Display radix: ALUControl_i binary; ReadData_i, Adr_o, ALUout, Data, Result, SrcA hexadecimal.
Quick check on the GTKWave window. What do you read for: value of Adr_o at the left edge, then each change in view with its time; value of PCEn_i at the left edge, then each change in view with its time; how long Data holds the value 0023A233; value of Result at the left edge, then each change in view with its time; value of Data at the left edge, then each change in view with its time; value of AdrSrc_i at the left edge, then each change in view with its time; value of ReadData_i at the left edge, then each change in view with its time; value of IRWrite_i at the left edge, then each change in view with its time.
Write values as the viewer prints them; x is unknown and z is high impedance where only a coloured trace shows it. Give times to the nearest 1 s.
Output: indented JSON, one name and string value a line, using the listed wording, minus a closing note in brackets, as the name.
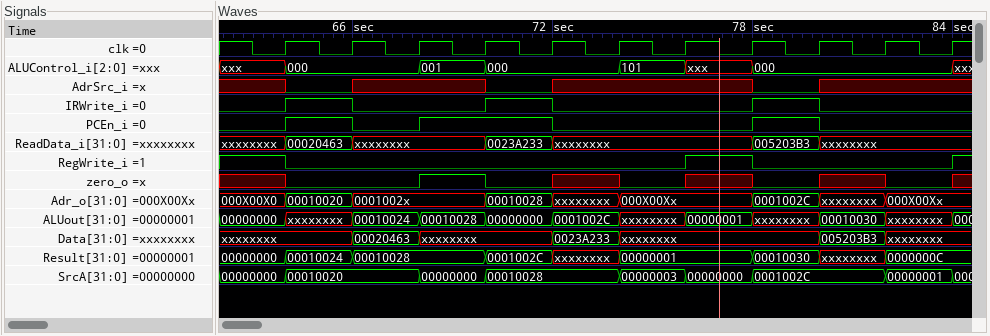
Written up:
{
  "value of Adr_o at the left edge, then each change in view with its time": "000X00X0, 00010020 at 64 s, 0001002x at 66 s, 00010028 at 70 s, xxxxxxxx at 72 s, 000X00Xx at 74 s, 0001002C at 78 s, xxxxxxxx at 80 s, 000X00Xx at 82 s",
  "value of PCEn_i at the left edge, then each change in view with its time": "0, 1 at 64 s, 0 at 66 s, 1 at 68 s, 0 at 72 s, 1 at 78 s, 0 at 80 s",
  "how long Data holds the value 0023A233": "2 s",
  "value of Result at the left edge, then each change in view with its time": "00000000, 00010024 at 64 s, 00010028 at 66 s, 0001002C at 70 s, xxxxxxxx at 72 s, 00000001 at 74 s, 00010030 at 78 s, xxxxxxxx at 80 s, 0000000C at 82 s",
  "value of Data at the left edge, then each change in view with its time": "xxxxxxxx, 00020463 at 66 s, xxxxxxxx at 68 s, 0023A233 at 72 s, xxxxxxxx at 74 s, 005203B3 at 80 s, xxxxxxxx at 82 s",
  "value of AdrSrc_i at the left edge, then each change in view with its time": "x, 0 at 64 s, x at 66 s, 0 at 70 s, x at 72 s, 0 at 78 s, x at 80 s",
  "value of ReadData_i at the left edge, then each change in view with its time": "xxxxxxxx, 00020463 at 64 s, xxxxxxxx at 66 s, 0023A233 at 70 s, xxxxxxxx at 72 s, 005203B3 at 78 s, xxxxxxxx at 80 s",
  "value of IRWrite_i at the left edge, then each change in view with its time": "0, 1 at 64 s, 0 at 66 s, 1 at 70 s, 0 at 72 s, 1 at 78 s, 0 at 80 s"
}
